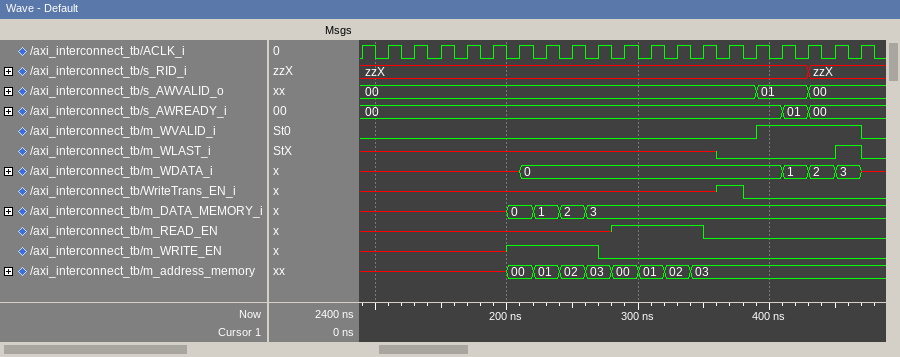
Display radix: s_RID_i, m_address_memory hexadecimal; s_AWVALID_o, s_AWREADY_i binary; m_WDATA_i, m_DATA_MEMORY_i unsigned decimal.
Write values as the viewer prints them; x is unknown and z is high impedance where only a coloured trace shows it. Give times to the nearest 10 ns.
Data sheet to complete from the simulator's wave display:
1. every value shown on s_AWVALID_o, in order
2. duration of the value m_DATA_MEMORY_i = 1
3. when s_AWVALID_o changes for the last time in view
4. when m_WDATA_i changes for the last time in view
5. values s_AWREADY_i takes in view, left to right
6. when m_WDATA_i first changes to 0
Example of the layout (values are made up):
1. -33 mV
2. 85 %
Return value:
1. 00, 01, 00
2. 20 ns
3. 430 ns
4. 470 ns
5. 00, 01, 00
6. 210 ns
